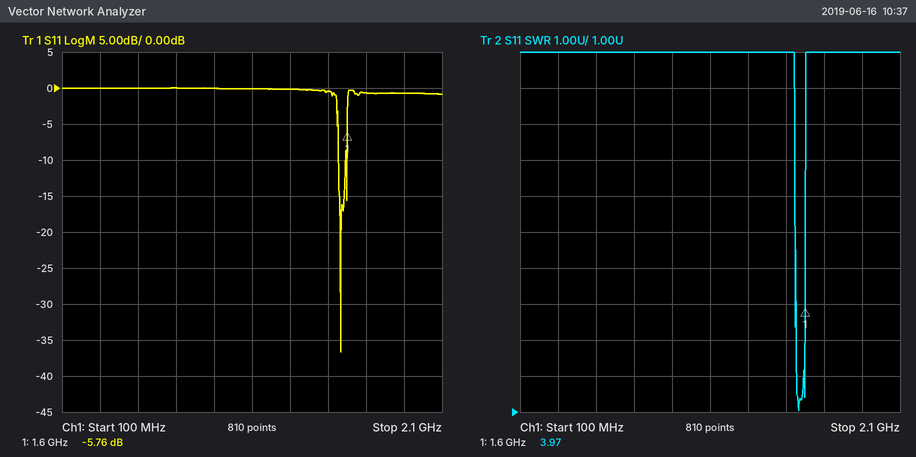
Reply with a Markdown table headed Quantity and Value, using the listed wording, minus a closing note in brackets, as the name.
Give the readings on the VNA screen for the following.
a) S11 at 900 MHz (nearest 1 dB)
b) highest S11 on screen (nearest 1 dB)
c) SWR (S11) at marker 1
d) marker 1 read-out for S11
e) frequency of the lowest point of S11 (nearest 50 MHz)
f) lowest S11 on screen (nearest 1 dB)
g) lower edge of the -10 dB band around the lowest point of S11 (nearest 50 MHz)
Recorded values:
| Quantity | Value |
|---|---|
| S11 at 900 MHz | 0 dB |
| highest S11 on screen | 0 dB |
| SWR (S11) at marker 1 | 3.97 |
| marker 1 read-out for S11 | -5.76 dB |
| frequency of the lowest point of S11 | 1.55 GHz |
| lowest S11 on screen | -37 dB |
| lower edge of the -10 dB band around the lowest point of S11 | 1.55 GHz |
